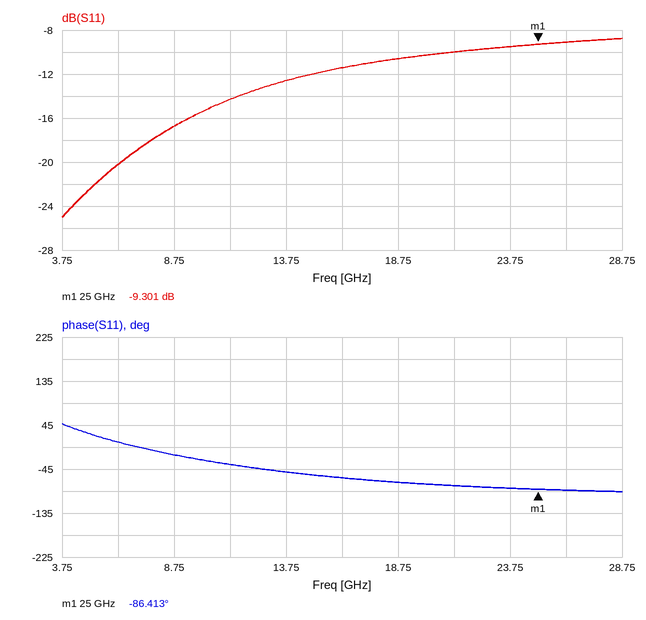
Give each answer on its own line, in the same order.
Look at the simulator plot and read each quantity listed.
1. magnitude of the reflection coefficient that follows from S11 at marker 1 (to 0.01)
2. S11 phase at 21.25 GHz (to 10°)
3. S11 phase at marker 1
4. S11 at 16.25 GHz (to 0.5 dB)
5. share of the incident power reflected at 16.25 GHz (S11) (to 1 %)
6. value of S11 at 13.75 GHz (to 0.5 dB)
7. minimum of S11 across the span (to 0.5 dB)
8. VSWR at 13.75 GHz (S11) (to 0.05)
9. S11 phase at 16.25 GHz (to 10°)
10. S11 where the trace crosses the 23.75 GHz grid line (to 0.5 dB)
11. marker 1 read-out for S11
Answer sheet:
0.34
-80°
-86.413°
-11.5 dB
7 %
-12.5 dB
-25.0 dB
1.60
-60°
-9.5 dB
-9.301 dB
